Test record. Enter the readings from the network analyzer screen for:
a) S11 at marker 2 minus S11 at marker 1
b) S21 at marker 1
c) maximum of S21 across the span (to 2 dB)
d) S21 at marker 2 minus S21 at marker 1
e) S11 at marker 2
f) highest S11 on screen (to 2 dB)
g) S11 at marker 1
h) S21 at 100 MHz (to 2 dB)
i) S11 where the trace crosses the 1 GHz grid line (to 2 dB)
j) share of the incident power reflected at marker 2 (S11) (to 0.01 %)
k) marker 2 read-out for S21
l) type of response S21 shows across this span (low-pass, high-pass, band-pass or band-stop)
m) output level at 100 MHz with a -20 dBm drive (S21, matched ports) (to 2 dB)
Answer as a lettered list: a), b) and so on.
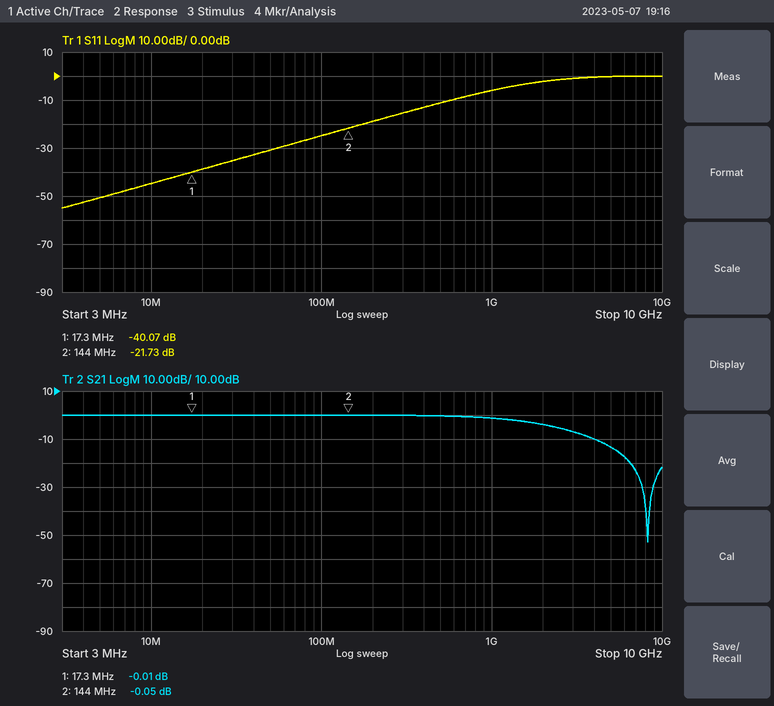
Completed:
a) 18.34 dB
b) -0.01 dB
c) 0 dB
d) -0.04 dB
e) -21.73 dB
f) 0 dB
g) -40.07 dB
h) 0 dB
i) -6 dB
j) 0.67 %
k) -0.05 dB
l) low-pass
m) -20 dBm
